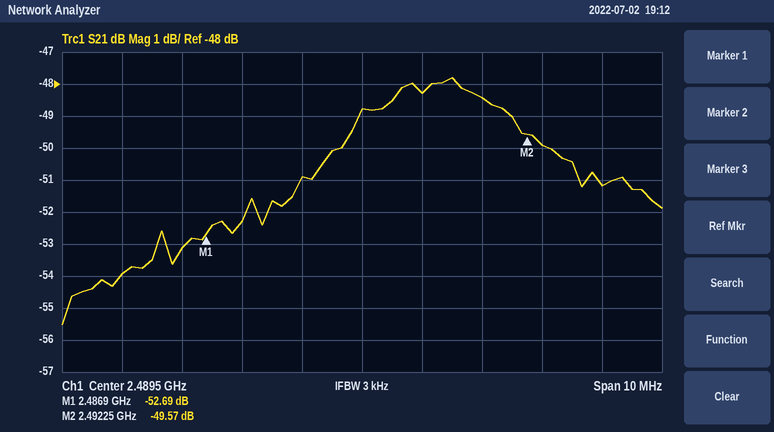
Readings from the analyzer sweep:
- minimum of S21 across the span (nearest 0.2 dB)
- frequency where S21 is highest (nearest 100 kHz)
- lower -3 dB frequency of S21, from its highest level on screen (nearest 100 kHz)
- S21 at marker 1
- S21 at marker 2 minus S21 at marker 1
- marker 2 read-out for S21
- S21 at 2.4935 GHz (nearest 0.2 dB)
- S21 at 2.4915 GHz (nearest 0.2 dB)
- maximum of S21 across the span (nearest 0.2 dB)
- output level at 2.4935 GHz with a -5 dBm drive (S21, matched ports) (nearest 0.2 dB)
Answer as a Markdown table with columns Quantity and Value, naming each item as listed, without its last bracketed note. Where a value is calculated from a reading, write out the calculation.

| Quantity | Value |
|---|---|
| minimum of S21 across the span | -55.6 dB |
| frequency where S21 is highest | 2.4910 GHz |
| lower -3 dB frequency of S21, from its highest level on screen | 2.4887 GHz |
| S21 at marker 1 | -52.69 dB |
| S21 at marker 2 minus S21 at marker 1 | -49.57 − (-52.69) = 3.12 dB |
| marker 2 read-out for S21 | -49.57 dB |
| S21 at 2.4935 GHz | -51.2 dB |
| S21 at 2.4915 GHz | -48.4 dB |
| maximum of S21 across the span | -47.8 dB |
| output level at 2.4935 GHz with a -5 dBm drive (S21, matched ports) | -5 dBm + (-51.2 dB) = -56.2 dBm |
